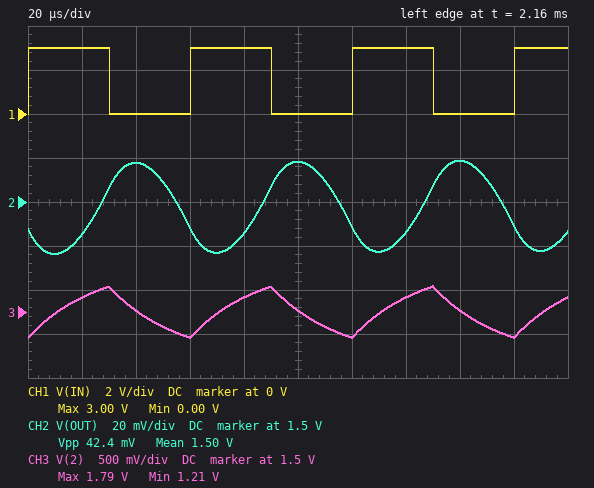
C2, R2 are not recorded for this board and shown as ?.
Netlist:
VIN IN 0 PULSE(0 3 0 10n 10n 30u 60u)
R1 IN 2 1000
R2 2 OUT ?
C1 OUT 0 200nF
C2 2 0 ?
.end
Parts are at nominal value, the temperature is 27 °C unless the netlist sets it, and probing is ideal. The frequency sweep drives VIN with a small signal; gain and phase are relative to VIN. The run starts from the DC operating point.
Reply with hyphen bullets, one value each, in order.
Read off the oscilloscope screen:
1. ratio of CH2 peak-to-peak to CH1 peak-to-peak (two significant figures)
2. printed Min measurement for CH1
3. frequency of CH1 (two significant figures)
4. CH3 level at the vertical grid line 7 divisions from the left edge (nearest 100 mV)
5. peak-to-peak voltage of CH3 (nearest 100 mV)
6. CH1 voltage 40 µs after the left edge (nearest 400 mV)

- 0.014
- 0.00 V
- 17 kHz
- 1.7 V
- 600 mV
- 0 V
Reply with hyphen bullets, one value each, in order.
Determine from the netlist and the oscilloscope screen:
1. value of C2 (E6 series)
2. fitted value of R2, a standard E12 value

- 68 nF
- 560 Ω
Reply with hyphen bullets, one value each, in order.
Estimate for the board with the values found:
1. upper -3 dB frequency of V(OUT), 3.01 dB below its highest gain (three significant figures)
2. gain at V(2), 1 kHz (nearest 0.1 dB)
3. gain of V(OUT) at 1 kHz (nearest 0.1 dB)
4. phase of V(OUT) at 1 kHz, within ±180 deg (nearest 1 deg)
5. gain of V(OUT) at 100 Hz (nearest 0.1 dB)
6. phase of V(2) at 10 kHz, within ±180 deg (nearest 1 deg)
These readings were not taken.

- 442 Hz
- -6.2 dB
- -7.9 dB
- -74 deg
- -0.2 dB
- -59 deg
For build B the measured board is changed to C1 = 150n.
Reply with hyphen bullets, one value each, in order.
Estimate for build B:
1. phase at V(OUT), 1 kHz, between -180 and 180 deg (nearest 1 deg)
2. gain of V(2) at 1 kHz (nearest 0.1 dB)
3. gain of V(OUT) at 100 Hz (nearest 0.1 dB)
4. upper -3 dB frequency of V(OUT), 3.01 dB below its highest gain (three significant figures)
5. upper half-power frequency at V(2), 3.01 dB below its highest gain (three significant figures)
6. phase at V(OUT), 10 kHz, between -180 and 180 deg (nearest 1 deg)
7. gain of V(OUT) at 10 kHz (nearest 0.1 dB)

- -68 deg
- -5.2 dB
- -0.1 dB
- 562 Hz
- 619 Hz
- -139 deg
- -29.2 dB
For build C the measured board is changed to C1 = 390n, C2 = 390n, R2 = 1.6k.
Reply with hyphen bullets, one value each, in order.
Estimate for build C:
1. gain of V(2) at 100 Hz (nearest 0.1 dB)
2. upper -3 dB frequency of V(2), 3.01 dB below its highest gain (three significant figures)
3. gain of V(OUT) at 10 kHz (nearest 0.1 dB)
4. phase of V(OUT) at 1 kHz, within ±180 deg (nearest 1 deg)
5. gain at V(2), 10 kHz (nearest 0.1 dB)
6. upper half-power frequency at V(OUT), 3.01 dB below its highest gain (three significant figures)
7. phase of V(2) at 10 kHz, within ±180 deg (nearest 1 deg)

- -1.4 dB
- 180 Hz
- -59.7 dB
- -134 deg
- -27.8 dB
- 129 Hz
- -86 deg
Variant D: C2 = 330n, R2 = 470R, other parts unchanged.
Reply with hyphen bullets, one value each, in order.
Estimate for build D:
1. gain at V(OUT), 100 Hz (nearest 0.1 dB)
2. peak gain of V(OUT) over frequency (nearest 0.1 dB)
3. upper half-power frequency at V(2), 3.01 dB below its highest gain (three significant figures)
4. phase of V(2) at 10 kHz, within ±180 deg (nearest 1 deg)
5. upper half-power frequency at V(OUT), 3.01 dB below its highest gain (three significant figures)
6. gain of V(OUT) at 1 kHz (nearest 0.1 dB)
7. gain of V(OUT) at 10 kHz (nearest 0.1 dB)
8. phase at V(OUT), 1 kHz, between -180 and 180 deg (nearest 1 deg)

- -0.5 dB
- 0 dB
- 285 Hz
- -82 deg
- 277 Hz
- -11.9 dB
- -42.1 dB
- -93 deg
